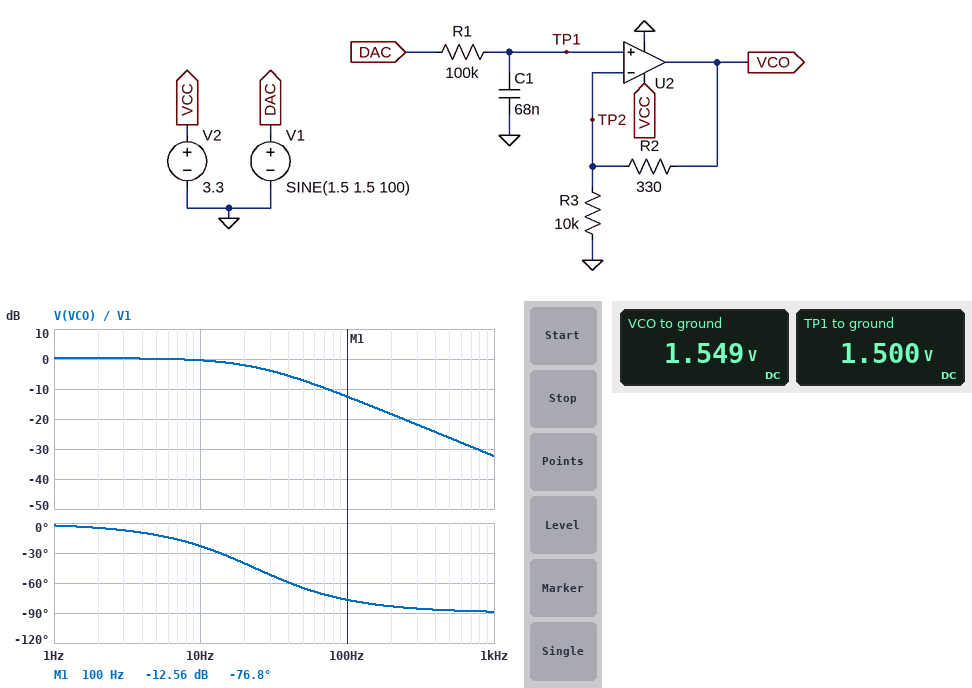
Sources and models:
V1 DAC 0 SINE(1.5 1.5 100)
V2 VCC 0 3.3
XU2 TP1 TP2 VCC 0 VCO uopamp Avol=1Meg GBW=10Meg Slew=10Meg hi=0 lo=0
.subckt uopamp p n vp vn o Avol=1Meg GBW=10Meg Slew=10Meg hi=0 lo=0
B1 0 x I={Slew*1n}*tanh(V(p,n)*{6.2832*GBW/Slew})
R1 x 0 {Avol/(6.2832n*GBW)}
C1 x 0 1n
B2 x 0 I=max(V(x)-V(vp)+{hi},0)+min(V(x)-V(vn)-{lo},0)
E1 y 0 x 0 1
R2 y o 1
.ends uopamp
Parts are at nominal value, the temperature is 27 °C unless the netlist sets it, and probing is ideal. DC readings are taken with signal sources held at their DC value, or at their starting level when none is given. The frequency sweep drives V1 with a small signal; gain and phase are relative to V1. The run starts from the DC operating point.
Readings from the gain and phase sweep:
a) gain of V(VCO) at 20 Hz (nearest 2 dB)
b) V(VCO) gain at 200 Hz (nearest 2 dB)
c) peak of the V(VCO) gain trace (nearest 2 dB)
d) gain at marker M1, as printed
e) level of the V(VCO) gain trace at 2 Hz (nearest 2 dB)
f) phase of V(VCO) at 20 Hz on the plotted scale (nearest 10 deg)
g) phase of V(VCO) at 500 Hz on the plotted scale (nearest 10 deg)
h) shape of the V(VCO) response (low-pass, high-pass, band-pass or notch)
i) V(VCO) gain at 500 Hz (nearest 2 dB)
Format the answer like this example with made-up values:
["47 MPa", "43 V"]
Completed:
["-2 dB", "-18 dB", "0 dB", "-12.56 dB", "0 dB", "-40 deg", "-90 deg", "low-pass", "-26 dB"]
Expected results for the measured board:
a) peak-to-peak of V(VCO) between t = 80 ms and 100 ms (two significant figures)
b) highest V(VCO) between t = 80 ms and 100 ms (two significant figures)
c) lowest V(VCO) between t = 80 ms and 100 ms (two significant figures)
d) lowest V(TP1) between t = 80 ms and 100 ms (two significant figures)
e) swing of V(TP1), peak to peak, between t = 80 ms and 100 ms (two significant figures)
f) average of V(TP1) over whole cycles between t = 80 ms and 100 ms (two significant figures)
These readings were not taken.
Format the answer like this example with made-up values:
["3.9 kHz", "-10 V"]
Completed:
["710 mV", "1.9 V", "1.2 V", "1.2 V", "680 mV", "1.5 V"]
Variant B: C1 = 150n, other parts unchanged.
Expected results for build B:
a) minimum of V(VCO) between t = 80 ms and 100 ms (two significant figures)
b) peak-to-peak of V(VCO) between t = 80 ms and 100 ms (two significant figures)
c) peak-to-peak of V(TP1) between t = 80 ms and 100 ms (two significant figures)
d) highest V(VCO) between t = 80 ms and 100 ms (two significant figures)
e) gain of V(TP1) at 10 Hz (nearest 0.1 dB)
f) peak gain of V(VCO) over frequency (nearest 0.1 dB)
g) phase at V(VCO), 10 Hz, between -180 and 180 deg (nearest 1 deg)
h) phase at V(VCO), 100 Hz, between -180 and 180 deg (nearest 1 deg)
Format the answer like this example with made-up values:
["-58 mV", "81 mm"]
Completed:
["1.4 V", "330 mV", "320 mV", "1.7 V", "-2.8 dB", "0.3 dB", "-43 deg", "-84 deg"]
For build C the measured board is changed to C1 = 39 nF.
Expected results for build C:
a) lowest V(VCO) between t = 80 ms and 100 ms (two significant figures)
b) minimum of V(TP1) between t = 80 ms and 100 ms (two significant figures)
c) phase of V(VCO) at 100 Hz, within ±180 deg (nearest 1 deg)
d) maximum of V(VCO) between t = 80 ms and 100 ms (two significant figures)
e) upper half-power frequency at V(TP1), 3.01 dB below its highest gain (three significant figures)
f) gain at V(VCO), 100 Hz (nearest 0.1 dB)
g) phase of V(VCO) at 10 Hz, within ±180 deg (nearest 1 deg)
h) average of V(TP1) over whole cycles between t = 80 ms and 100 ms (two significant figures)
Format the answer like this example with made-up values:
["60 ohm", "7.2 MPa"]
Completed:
["960 mV", "930 mV", "-68 deg", "2.1 V", "40.8 Hz", "-8.2 dB", "-14 deg", "1.5 V"]
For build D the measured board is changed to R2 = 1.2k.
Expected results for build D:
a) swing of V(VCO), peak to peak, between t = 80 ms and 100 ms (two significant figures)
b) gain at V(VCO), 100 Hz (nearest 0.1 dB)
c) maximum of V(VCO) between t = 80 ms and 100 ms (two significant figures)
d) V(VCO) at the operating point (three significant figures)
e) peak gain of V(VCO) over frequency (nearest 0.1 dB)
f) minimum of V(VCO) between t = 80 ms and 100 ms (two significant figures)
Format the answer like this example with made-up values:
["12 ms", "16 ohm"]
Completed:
["770 mV", "-11.9 dB", "2.1 V", "1.68 V", "1.0 dB", "1.3 V"]
